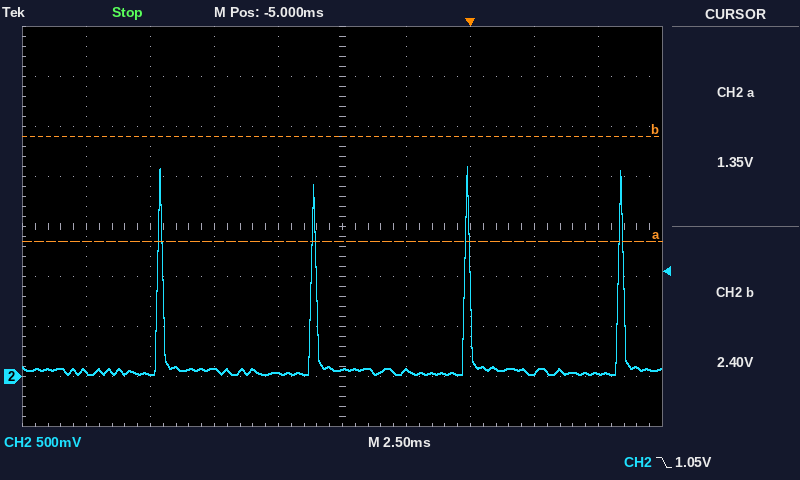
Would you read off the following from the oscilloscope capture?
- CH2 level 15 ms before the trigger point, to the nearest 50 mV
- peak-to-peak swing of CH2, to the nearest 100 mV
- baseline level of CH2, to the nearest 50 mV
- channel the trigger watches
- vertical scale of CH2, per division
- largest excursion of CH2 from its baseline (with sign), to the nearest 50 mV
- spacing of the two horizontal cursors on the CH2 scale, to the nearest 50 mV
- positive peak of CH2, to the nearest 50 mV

50 mV
2.10 V
50 mV
CH2
500 mV
+2.05 V
1.05 V
2.10 V
